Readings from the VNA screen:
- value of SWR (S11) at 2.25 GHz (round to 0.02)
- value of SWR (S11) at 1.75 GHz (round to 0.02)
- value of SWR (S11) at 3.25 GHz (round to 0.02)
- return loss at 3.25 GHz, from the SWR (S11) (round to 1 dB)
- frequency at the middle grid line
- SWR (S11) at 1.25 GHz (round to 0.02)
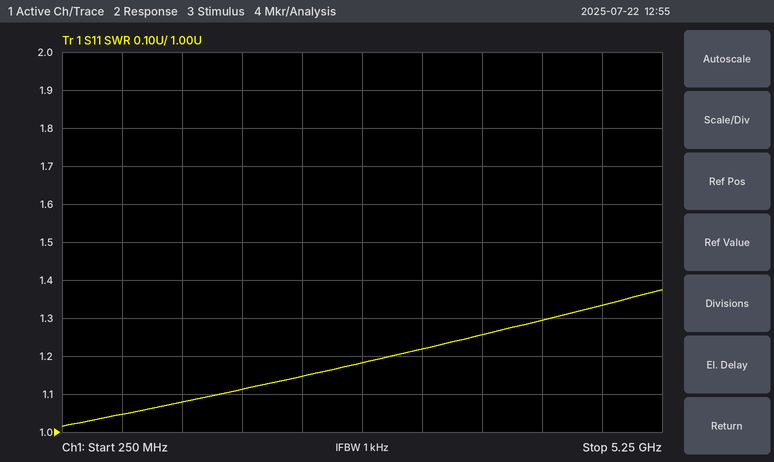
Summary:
1.14
1.12
1.22
20 dB
2.75 GHz
1.08
